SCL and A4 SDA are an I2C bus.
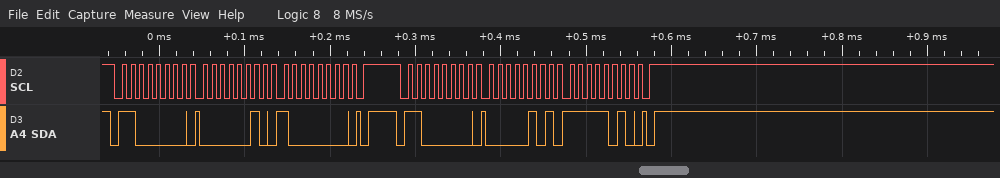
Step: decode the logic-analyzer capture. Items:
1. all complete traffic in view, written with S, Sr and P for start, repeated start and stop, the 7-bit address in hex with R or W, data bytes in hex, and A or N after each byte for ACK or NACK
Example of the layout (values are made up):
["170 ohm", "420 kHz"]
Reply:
["S 60W A 02 A 80 A P S 60W A 05 A FA A P"]
